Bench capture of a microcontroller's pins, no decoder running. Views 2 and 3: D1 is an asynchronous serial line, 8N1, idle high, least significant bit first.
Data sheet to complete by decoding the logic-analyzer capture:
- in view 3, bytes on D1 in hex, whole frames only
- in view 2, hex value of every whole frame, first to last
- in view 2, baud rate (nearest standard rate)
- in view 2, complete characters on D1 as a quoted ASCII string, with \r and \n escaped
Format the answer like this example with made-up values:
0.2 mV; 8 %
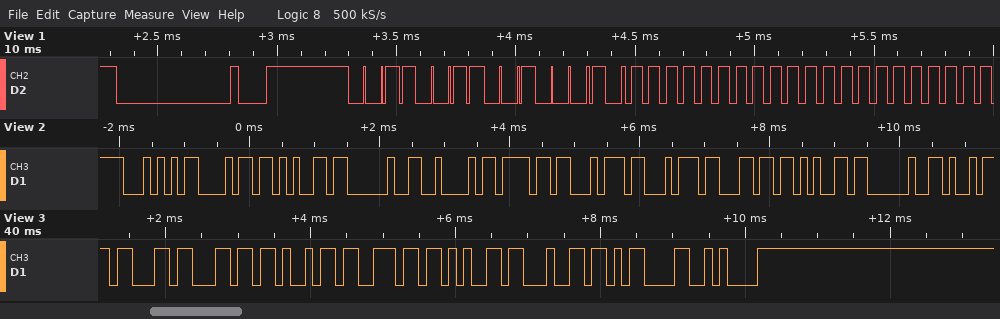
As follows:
0x63 0x6C 0x69 0x6E 0x65 0x64 0x0D 0x0A; 0x54 0x68 0x65 0x20 0x42 0x6F 0x74 0x74 0x6C 0x65 0x20; 9600 baud; "The Bottle "
